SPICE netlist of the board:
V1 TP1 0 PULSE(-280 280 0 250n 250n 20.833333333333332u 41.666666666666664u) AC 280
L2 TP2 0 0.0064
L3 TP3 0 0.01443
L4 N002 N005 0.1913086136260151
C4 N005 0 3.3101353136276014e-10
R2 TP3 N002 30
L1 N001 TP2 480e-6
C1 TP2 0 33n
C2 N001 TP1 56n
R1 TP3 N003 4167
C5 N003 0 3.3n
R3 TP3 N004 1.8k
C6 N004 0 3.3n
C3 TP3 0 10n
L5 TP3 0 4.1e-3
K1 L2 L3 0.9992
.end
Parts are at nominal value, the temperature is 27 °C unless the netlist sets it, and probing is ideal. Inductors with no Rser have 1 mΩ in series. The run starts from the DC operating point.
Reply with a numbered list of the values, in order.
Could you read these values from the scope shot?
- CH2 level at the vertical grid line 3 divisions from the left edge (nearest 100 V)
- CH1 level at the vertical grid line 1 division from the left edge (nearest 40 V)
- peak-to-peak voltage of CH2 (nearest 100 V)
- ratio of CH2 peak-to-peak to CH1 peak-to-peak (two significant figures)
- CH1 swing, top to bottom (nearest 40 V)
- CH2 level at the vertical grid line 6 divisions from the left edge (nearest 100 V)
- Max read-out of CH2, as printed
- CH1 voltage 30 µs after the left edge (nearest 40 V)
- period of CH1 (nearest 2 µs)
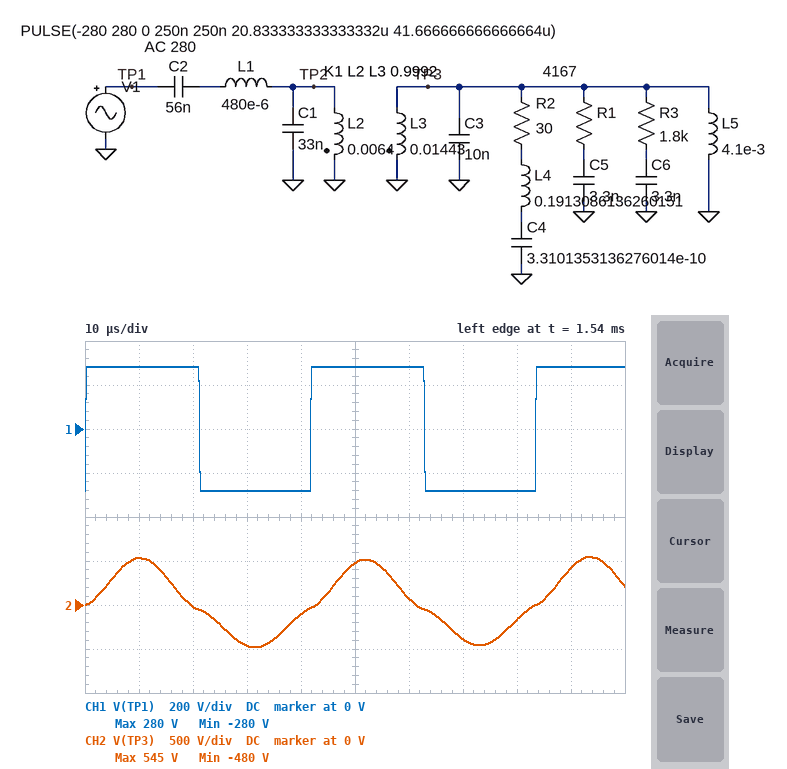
1. -500 V
2. 280 V
3. 1.0 kV
4. 1.8
5. 560 V
6. 100 V
7. 545 V
8. -280 V
9. 42 µs
